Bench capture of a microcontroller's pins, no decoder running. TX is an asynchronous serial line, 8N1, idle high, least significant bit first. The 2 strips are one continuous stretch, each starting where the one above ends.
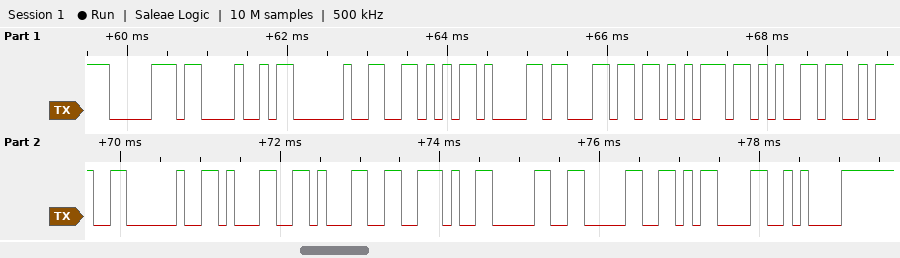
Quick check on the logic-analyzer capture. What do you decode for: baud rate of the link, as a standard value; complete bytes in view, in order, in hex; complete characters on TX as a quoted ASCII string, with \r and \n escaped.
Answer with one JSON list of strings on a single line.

["9600 baud", "0x70 0x48 0x20 0x56 0x61 0x6C 0x75 0x65 0x3A 0x20 0x31 0x31 0x2E 0x30 0x30 0x0D 0x0A", "\"pH Value: 11.00\\r\\n\""]
